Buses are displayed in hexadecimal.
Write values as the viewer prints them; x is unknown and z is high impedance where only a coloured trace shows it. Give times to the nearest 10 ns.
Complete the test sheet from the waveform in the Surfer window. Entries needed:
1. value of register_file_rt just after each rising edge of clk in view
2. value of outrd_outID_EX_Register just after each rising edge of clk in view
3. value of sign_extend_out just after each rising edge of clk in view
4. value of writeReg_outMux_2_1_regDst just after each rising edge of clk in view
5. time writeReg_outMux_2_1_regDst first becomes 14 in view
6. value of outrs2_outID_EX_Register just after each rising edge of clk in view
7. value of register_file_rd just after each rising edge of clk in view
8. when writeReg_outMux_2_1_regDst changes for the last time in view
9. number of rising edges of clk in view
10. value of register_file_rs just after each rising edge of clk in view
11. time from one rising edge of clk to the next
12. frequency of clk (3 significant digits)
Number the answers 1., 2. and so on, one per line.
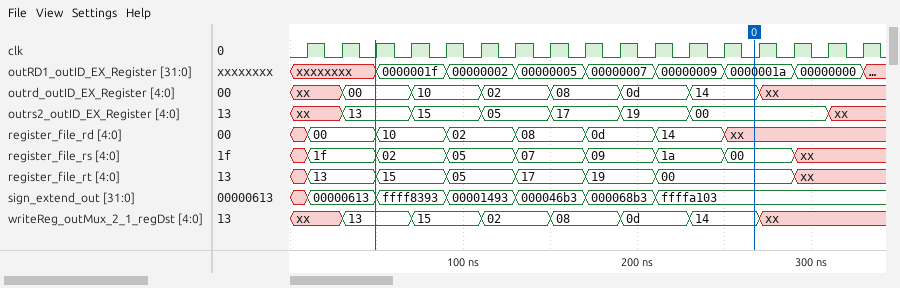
1. 13, 13, 15, 15, 05, 05, 17, 17, 19, 19, 00, 00, 00, 00, xx, xx, xx
2. xx, 00, 00, 10, 10, 02, 02, 08, 08, 0d, 0d, 14, 14, xx, xx, xx, xx
3. 00000613, 00000613, ffff8393, ffff8393, 00001493, 00001493, 000046b3, 000046b3, 000068b3, 000068b3, ffffa103, ffffa103, ffffa103, ffffa103, ffffa103, ffffa103, ffffa103
4. xx, 13, 13, 15, 15, 02, 02, 08, 08, 0d, 0d, 14, 14, xx, xx, xx, xx
5. 230 ns
6. xx, 13, 13, 15, 15, 05, 05, 17, 17, 19, 19, 00, 00, 00, 00, xx, xx
7. 00, 00, 10, 10, 02, 02, 08, 08, 0d, 0d, 14, 14, xx, xx, xx, xx, xx
8. 270 ns
9. 17
10. 1f, 1f, 02, 02, 05, 05, 07, 07, 09, 09, 1a, 1a, 00, 00, xx, xx, xx
11. 20 ns
12. 50.0 MHz
